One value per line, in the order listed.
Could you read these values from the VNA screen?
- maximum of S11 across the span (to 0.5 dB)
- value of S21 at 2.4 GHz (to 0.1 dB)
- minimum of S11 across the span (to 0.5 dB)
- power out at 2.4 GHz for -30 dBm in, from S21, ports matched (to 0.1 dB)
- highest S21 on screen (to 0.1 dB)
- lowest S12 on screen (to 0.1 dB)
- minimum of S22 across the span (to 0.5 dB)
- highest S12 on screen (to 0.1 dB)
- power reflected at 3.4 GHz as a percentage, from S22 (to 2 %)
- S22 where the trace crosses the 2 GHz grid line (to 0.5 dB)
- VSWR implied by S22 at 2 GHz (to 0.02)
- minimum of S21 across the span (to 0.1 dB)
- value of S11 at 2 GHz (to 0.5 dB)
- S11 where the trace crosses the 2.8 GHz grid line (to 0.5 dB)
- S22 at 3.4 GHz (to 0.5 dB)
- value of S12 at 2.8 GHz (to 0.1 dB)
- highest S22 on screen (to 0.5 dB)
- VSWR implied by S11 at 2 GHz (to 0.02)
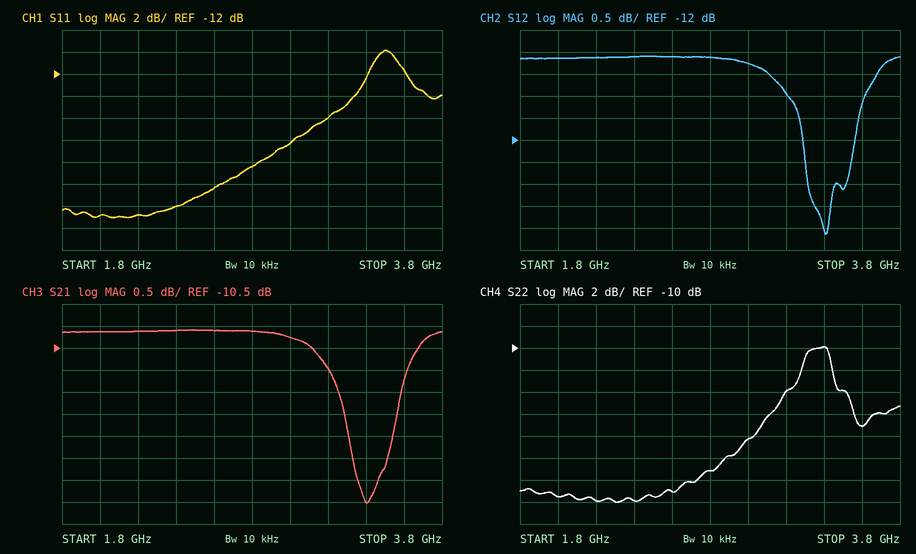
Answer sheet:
-10.0 dB
-10.1 dB
-25.0 dB
-40.1 dBm
-10.1 dB
-14.1 dB
-24.0 dB
-10.1 dB
10 %
-23.5 dB
1.14
-14.0 dB
-25.0 dB
-20.5 dB
-10.0 dB
-10.1 dB
-10.0 dB
1.12
